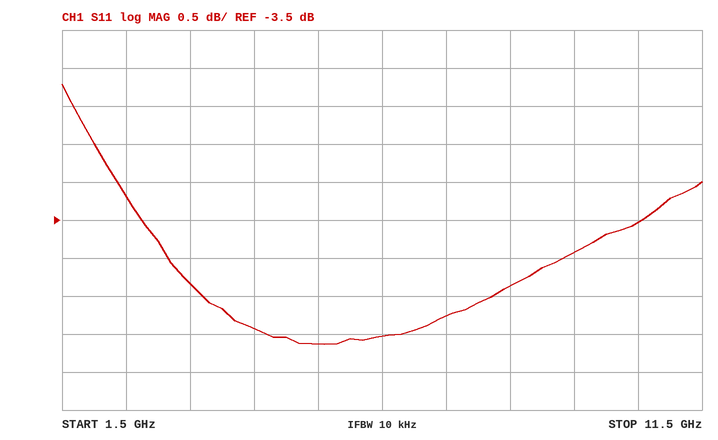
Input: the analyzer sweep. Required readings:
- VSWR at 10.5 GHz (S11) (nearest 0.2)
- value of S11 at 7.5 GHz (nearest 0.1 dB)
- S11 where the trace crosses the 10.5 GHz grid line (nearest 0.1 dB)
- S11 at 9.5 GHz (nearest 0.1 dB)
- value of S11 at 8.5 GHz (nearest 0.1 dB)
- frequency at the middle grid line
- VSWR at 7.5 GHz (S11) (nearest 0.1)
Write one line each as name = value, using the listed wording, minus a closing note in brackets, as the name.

VSWR at 10.5 GHz (S11) = 5.0
value of S11 at 7.5 GHz = -4.8 dB
S11 where the trace crosses the 10.5 GHz grid line = -3.5 dB
S11 at 9.5 GHz = -3.9 dB
value of S11 at 8.5 GHz = -4.4 dB
frequency at the middle grid line = 6.5 GHz
VSWR at 7.5 GHz (S11) = 3.7
